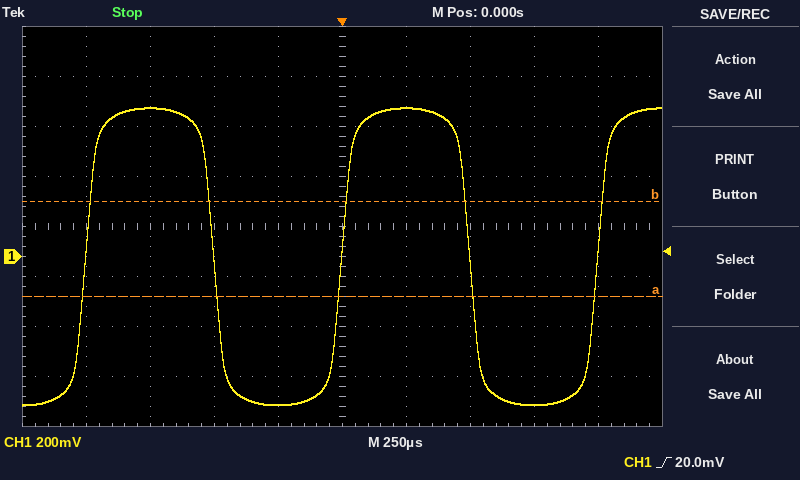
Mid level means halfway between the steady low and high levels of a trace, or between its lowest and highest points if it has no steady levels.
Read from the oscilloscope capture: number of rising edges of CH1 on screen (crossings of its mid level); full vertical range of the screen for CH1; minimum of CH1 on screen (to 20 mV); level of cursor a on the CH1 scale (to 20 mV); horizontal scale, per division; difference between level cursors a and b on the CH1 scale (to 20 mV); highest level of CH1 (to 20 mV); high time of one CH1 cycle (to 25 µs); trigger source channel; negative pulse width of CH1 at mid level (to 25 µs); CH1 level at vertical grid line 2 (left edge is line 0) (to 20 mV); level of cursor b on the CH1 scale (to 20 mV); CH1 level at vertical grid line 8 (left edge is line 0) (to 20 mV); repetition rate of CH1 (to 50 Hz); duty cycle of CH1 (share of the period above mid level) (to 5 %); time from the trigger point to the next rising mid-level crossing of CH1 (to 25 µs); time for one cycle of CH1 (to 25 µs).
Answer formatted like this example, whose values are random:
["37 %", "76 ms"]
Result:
["3", "1.6 V", "-600 mV", "-160 mV", "250 µs", "380 mV", "600 mV", "500 µs", "CH1", "500 µs", "600 mV", "220 mV", "-600 mV", "1.00 kHz", "50 %", "1.000 ms", "1.000 ms"]
